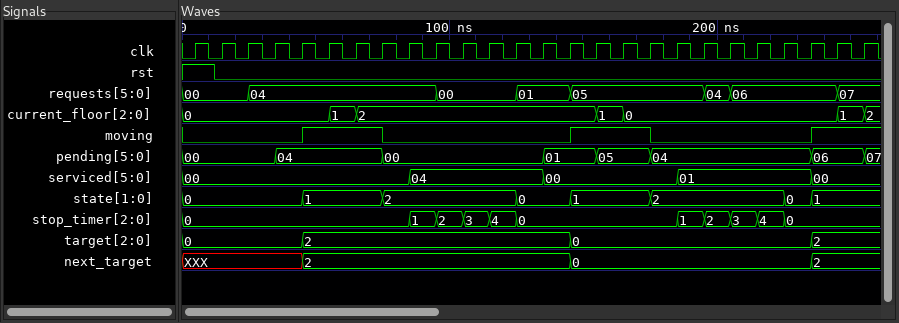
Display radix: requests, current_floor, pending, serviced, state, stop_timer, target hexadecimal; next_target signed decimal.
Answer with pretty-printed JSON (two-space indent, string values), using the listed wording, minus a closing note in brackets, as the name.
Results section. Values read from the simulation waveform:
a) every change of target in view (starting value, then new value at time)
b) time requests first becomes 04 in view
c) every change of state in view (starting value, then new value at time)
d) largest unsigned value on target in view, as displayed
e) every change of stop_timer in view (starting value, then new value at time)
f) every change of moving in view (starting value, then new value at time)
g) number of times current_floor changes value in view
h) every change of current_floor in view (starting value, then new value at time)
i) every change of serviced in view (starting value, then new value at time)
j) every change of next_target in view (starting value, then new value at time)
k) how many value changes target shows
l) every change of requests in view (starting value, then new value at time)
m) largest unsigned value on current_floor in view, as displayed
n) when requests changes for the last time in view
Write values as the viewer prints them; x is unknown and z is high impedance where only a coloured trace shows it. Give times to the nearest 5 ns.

{
  "every change of target in view": "0, 2 at 45 ns, 0 at 145 ns, 2 at 235 ns",
  "time requests first becomes 04 in view": "25 ns",
  "every change of state in view": "0, 1 at 45 ns, 2 at 75 ns, 0 at 125 ns, 1 at 145 ns, 2 at 175 ns, 0 at 225 ns, 1 at 235 ns",
  "largest unsigned value on target in view, as displayed": "2",
  "every change of stop_timer in view": "0, 1 at 85 ns, 2 at 95 ns, 3 at 105 ns, 4 at 115 ns, 0 at 125 ns, 1 at 185 ns, 2 at 195 ns, 3 at 205 ns, 4 at 215 ns, 0 at 225 ns",
  "every change of moving in view": "0, 1 at 45 ns, 0 at 75 ns, 1 at 145 ns, 0 at 175 ns, 1 at 235 ns",
  "number of times current_floor changes value in view": "6",
  "every change of current_floor in view": "0, 1 at 55 ns, 2 at 65 ns, 1 at 155 ns, 0 at 165 ns, 1 at 245 ns, 2 at 255 ns",
  "every change of serviced in view": "00, 04 at 85 ns, 00 at 135 ns, 01 at 185 ns, 00 at 235 ns",
  "every change of next_target in view": "XXX, 2 at 45 ns, 0 at 145 ns, 2 at 235 ns",
  "how many value changes target shows": "3",
  "every change of requests in view": "00, 04 at 25 ns, 00 at 95 ns, 01 at 125 ns, 05 at 145 ns, 04 at 195 ns, 06 at 205 ns, 07 at 245 ns",
  "largest unsigned value on current_floor in view, as displayed": "2",
  "when requests changes for the last time in view": "245 ns"
}
